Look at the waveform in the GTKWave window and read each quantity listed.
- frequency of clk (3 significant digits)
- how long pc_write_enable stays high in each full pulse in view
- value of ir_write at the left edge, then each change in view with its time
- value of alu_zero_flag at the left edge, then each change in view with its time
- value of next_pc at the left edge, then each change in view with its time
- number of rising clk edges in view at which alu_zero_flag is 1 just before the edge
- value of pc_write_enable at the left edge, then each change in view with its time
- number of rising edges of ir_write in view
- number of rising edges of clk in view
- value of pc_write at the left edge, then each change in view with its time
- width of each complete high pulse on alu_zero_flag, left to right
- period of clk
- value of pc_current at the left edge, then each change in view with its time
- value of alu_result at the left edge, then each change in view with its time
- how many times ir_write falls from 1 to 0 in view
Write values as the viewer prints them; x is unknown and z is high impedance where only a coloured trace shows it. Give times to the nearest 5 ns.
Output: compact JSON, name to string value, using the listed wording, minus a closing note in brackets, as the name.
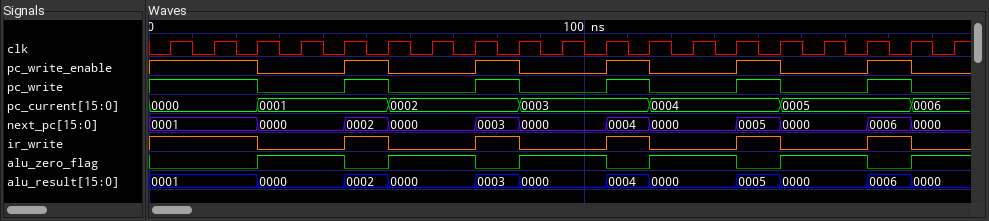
{"frequency of clk": "100 MHz", "how long pc_write_enable stays high in each full pulse in view": "10 ns, 10 ns, 10 ns, 10 ns, 10 ns", "value of ir_write at the left edge, then each change in view with its time": "1, 0 at 25 ns, 1 at 45 ns, 0 at 55 ns, 1 at 75 ns, 0 at 85 ns, 1 at 105 ns, 0 at 115 ns, 1 at 135 ns, 0 at 145 ns, 1 at 165 ns, 0 at 175 ns", "value of alu_zero_flag at the left edge, then each change in view with its time": "0, 1 at 25 ns, 0 at 45 ns, 1 at 55 ns, 0 at 75 ns, 1 at 85 ns, 0 at 105 ns, 1 at 115 ns, 0 at 135 ns, 1 at 145 ns, 0 at 165 ns, 1 at 175 ns", "value of next_pc at the left edge, then each change in view with its time": "0001, 0000 at 25 ns, 0002 at 45 ns, 0000 at 55 ns, 0003 at 75 ns, 0000 at 85 ns, 0004 at 105 ns, 0000 at 115 ns, 0005 at 135 ns, 0000 at 145 ns, 0006 at 165 ns, 0000 at 175 ns", "number of rising clk edges in view at which alu_zero_flag is 1 just before the edge": "11", "value of pc_write_enable at the left edge, then each change in view with its time": "1, 0 at 25 ns, 1 at 45 ns, 0 at 55 ns, 1 at 75 ns, 0 at 85 ns, 1 at 105 ns, 0 at 115 ns, 1 at 135 ns, 0 at 145 ns, 1 at 165 ns, 0 at 175 ns", "number of rising edges of ir_write in view": "5", "number of rising edges of clk in view": "19", "value of pc_write at the left edge, then each change in view with its time": "1, 0 at 25 ns, 1 at 45 ns, 0 at 55 ns, 1 at 75 ns, 0 at 85 ns, 1 at 105 ns, 0 at 115 ns, 1 at 135 ns, 0 at 145 ns, 1 at 165 ns, 0 at 175 ns", "width of each complete high pulse on alu_zero_flag, left to right": "20 ns, 20 ns, 20 ns, 20 ns, 20 ns", "period of clk": "10 ns", "value of pc_current at the left edge, then each change in view with its time": "0000, 0001 at 25 ns, 0002 at 55 ns, 0003 at 85 ns, 0004 at 115 ns, 0005 at 145 ns, 0006 at 175 ns", "value of alu_result at the left edge, then each change in view with its time": "0001, 0000 at 25 ns, 0002 at 45 ns, 0000 at 55 ns, 0003 at 75 ns, 0000 at 85 ns, 0004 at 105 ns, 0000 at 115 ns, 0005 at 135 ns, 0000 at 145 ns, 0006 at 165 ns, 0000 at 175 ns", "how many times ir_write falls from 1 to 0 in view": "6"}
